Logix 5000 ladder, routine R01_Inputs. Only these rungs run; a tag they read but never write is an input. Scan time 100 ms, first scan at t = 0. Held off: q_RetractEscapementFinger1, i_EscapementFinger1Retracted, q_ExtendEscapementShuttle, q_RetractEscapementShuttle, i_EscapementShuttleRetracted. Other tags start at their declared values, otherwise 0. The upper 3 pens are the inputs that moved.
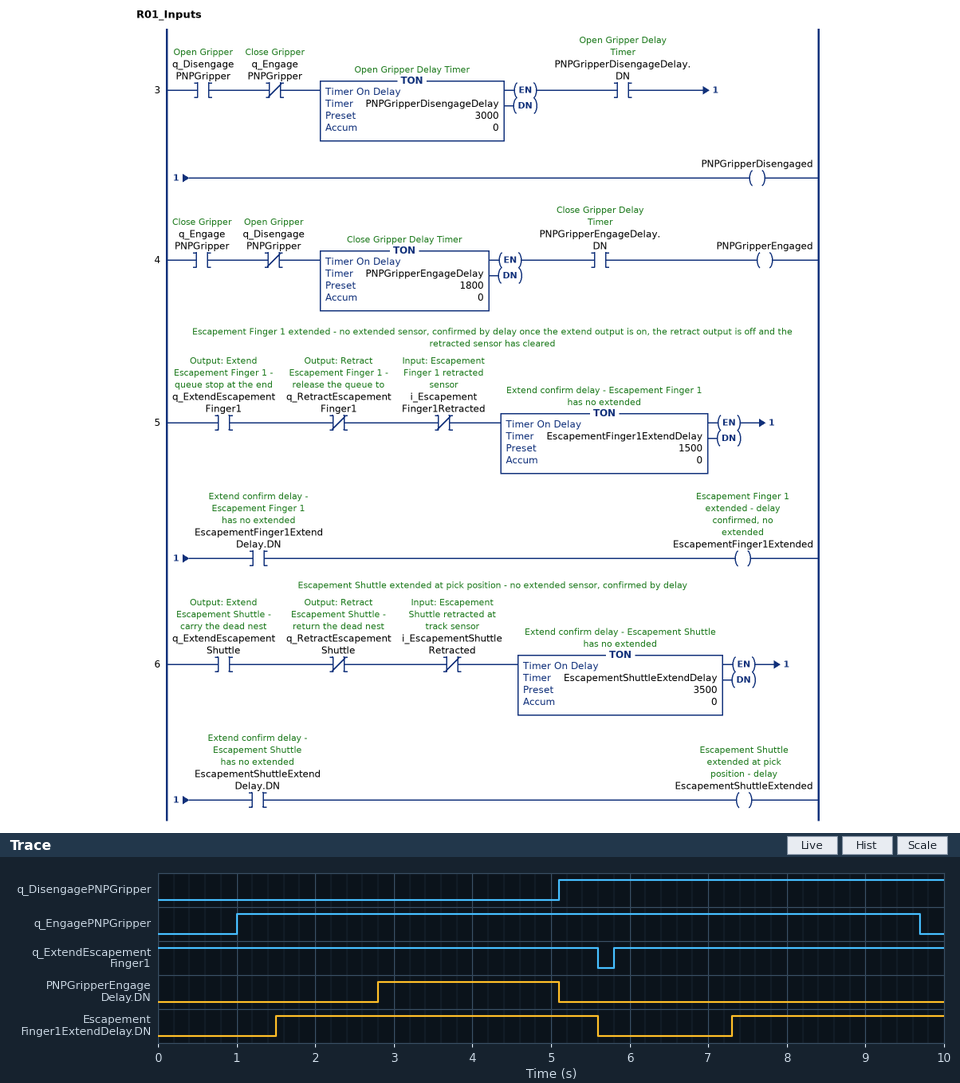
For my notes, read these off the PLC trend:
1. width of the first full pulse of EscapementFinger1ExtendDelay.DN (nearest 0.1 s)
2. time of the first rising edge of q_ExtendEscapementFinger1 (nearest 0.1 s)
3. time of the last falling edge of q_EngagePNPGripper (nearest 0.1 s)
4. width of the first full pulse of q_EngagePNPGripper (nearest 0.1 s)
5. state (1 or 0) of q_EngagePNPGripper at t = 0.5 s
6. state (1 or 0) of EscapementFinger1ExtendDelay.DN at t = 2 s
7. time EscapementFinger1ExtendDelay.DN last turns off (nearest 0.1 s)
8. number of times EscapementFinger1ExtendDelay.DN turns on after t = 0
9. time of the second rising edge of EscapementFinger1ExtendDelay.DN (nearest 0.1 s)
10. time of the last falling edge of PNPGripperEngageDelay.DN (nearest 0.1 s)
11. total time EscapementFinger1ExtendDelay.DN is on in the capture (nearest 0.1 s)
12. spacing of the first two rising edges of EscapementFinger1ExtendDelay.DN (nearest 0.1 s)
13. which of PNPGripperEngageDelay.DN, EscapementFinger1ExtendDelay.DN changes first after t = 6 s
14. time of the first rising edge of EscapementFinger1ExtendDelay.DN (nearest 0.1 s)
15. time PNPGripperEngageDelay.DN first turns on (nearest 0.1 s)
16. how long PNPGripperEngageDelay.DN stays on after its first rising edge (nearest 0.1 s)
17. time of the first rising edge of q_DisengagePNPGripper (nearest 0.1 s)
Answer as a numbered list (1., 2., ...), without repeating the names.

1. 4.1 s
2. 5.8 s
3. 9.7 s
4. 8.7 s
5. 0
6. 1
7. 5.6 s
8. 2
9. 7.3 s
10. 5.1 s
11. 6.8 s
12. 5.8 s
13. EscapementFinger1ExtendDelay.DN
14. 1.5 s
15. 2.8 s
16. 2.3 s
17. 5.1 s
